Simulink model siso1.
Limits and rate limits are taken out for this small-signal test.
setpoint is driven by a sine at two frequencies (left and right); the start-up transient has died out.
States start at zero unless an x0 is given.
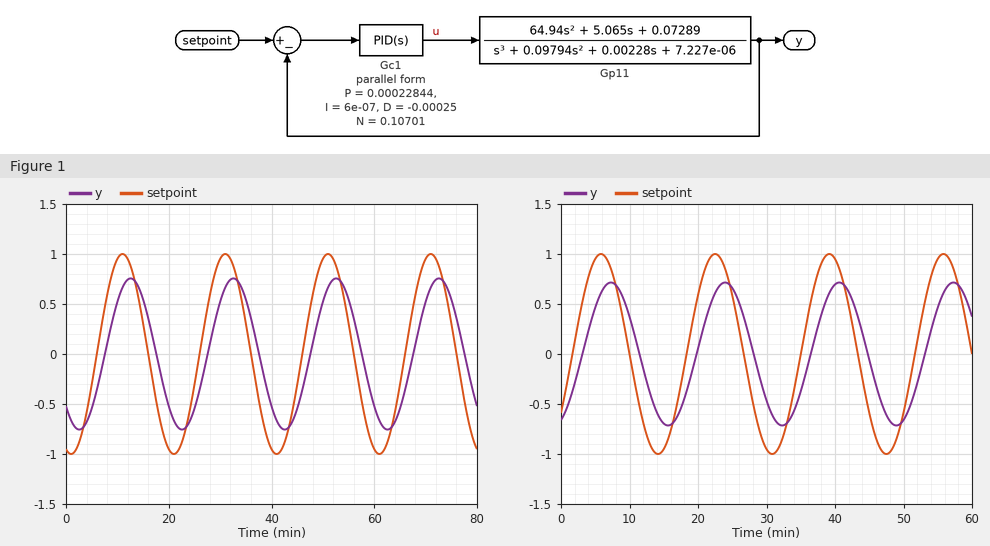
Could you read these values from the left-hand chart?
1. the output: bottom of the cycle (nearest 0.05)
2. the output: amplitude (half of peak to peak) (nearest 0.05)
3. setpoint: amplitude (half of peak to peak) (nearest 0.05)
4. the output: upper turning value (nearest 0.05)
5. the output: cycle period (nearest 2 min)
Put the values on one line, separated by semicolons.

-0.75; 0.75; 1.00; 0.75; 20 min
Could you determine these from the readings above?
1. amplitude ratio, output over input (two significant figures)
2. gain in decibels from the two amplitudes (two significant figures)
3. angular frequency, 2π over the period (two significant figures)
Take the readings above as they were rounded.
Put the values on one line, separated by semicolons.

0.75; -2.5 dB; 0.31 rad/min
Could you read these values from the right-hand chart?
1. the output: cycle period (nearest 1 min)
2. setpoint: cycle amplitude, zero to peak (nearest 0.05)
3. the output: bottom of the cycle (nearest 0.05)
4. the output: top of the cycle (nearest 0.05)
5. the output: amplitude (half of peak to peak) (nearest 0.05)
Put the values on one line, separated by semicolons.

17 min; 1.00; -0.70; 0.70; 0.70
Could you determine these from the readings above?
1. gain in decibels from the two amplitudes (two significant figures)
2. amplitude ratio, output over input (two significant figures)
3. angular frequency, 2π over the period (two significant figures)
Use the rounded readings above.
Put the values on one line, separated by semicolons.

-3.1 dB; 0.70; 0.37 rad/min
